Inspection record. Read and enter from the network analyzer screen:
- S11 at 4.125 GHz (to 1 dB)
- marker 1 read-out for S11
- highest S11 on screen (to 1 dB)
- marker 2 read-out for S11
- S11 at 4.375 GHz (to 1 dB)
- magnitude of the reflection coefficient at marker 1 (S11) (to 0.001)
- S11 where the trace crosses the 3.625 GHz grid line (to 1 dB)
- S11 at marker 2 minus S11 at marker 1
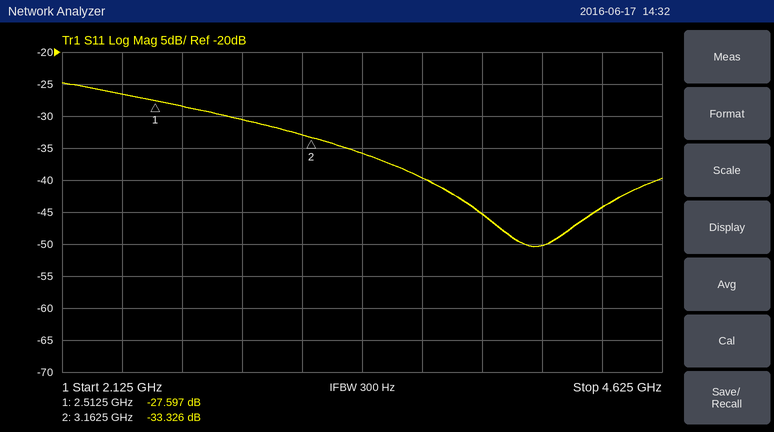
-50 dB
-27.597 dB
-25 dB
-33.326 dB
-44 dB
0.042
-40 dB
-5.729 dB
